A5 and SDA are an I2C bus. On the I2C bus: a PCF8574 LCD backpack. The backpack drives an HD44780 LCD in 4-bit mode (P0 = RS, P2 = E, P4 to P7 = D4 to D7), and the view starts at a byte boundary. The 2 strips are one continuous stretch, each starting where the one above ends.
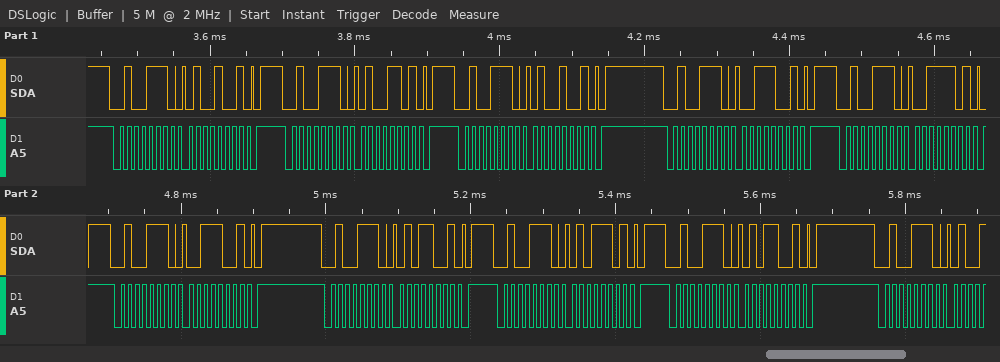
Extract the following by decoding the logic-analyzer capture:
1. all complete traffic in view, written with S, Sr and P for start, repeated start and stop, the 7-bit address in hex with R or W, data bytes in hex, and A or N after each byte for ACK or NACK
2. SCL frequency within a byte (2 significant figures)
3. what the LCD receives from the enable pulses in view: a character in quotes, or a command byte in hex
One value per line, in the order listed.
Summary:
S 27W A 49 A P S 27W A 4D A P S 27W A 49 A P S 27W A 39 A P S 27W A 3D A P S 27W A 39 A P S 27W A 59 A P S 27W A 5D A P S 27W A 59 A P S 27W A
100 kHz
'C'
